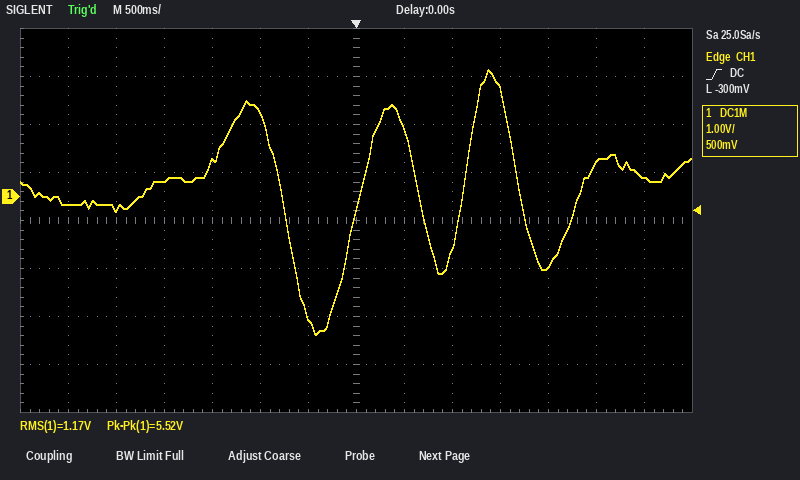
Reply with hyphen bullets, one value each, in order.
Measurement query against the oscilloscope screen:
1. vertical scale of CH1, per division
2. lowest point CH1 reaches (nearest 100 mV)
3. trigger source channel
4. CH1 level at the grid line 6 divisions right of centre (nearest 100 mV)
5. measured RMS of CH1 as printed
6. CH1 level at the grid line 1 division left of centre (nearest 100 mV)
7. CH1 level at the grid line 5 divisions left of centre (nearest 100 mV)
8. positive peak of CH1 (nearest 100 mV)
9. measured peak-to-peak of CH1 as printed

- 1 V
- -2.9 V
- CH1
- 400 mV
- 1.17 V
- -2.5 V
- -300 mV
- 2.6 V
- 5.52 V
